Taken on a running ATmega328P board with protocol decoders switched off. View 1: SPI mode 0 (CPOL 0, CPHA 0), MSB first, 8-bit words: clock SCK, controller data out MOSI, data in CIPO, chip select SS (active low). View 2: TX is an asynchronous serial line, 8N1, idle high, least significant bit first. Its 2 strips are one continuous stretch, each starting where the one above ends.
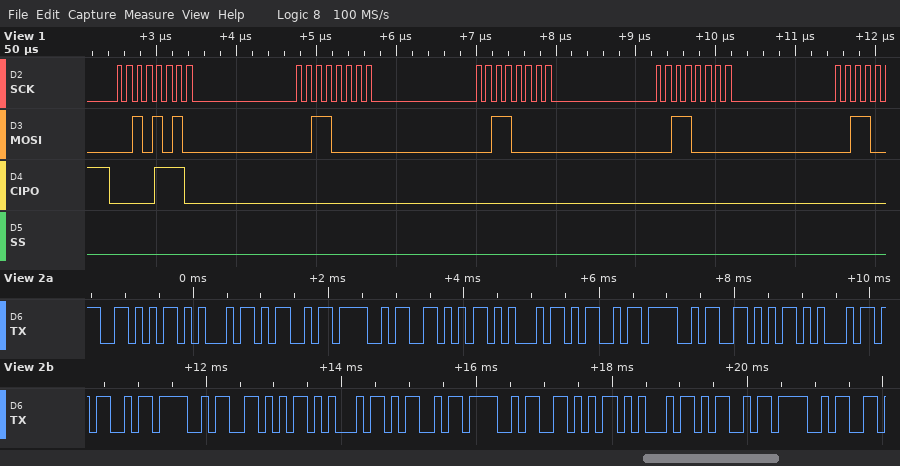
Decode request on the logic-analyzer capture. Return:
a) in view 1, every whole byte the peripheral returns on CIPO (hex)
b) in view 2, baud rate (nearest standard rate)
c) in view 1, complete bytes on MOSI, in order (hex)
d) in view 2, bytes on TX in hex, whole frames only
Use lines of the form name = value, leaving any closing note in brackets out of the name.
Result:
in view 1, every whole byte the peripheral returns on CIPO = 0E 00 00 00
in view 2, baud rate = 9600 baud
in view 1, complete bytes on MOSI, in order = 2A 30 30 30
in view 2, bytes on TX in hex, whole frames only = 56 45 4D 4F 56 45 4D 4F 56 45 4D 4F 56 45 4D 4F 56 45 4D 4F
